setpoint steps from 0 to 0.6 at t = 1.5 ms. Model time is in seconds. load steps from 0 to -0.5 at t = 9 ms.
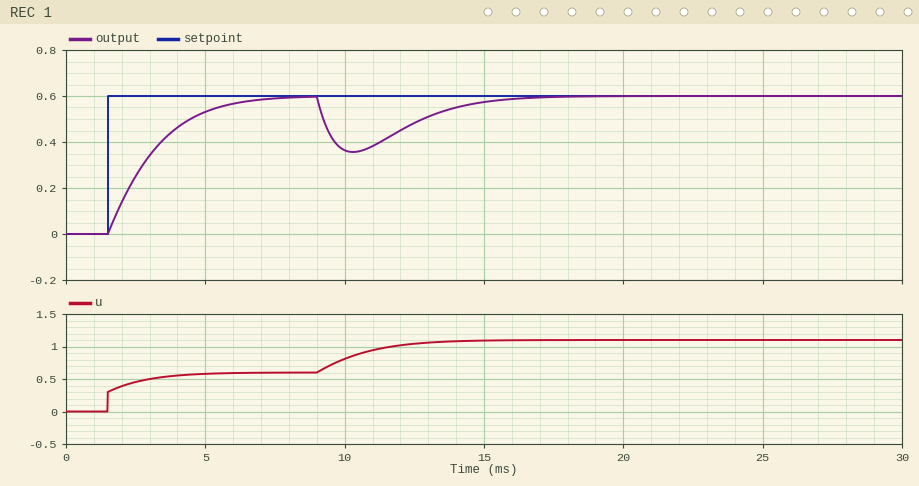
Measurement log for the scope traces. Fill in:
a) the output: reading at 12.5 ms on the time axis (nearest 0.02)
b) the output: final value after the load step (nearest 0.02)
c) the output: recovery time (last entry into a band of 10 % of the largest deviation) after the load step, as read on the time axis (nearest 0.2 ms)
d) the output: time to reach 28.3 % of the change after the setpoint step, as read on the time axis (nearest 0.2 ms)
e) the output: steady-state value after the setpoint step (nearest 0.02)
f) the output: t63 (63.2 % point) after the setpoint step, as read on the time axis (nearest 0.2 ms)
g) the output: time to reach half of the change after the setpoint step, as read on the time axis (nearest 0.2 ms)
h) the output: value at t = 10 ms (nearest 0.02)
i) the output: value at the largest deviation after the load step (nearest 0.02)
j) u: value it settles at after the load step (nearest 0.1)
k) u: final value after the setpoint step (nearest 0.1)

0.48
0.60
15.2 ms
2.2 ms
0.60
3.2 ms
2.8 ms
0.36
0.36
1.1
0.6
